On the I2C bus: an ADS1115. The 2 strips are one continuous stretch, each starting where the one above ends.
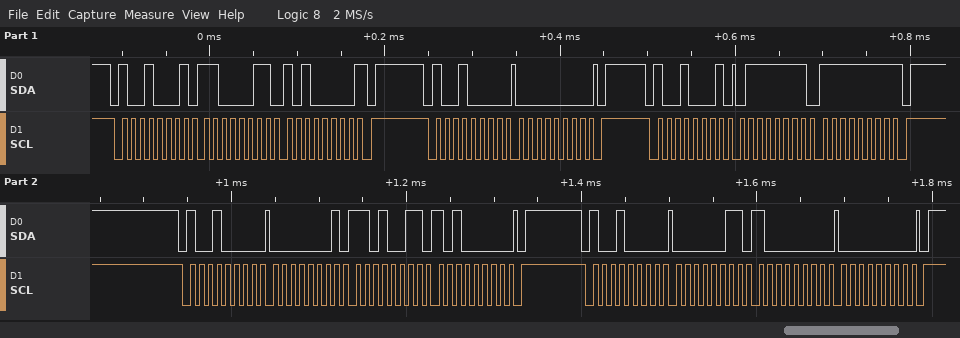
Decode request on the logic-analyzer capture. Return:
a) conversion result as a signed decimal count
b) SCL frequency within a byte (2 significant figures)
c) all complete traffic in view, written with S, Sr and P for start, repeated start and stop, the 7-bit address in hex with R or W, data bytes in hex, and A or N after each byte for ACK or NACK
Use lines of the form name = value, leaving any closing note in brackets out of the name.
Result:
conversion result as a signed decimal count = 32767
SCL frequency within a byte = 100 kHz
all complete traffic in view, written with S, Sr and P for start, repeated start and stop, the 7-bit address in hex with R or W, data bytes in hex, and A or N after each byte for ACK or NACK = S 48R A C3 A A0 N P S 48W A 00 A P S 48R A 7F A FF N P S 48W A 01 A D3 A A0 A P S 48W A 03 A 80 A 00 A P
